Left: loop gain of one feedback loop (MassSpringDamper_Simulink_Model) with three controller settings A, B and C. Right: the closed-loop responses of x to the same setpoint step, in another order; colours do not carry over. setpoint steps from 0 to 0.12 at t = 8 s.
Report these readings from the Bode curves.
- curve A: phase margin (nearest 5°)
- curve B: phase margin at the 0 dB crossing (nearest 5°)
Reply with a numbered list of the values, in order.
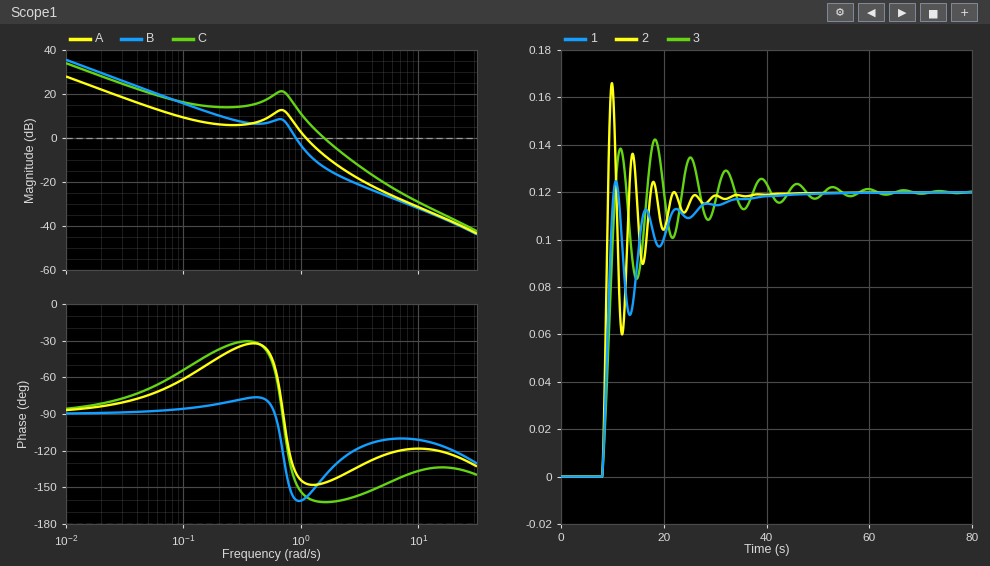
1. 35°
2. 20°
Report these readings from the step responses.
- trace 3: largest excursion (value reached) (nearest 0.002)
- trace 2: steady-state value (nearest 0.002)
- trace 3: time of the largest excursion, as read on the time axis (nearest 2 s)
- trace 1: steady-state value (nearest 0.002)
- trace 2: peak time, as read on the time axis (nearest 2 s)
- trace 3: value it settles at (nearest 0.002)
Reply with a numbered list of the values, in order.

1. 0.142
2. 0.120
3. 18 s
4. 0.120
5. 10 s
6. 0.120
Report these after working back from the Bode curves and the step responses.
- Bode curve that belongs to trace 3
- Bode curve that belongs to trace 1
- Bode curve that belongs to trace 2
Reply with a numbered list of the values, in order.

1. B
2. A
3. C
